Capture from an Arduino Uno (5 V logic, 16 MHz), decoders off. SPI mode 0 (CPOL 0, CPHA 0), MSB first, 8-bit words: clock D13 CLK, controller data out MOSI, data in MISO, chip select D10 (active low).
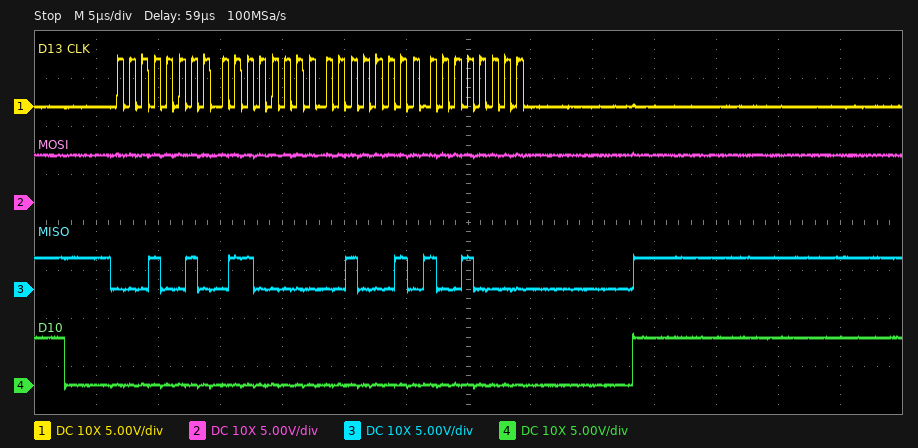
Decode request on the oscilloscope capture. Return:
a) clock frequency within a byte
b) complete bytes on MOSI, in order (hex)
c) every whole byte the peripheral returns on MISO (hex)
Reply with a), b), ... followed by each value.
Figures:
a) 1 MHz
b) 0xFF 0xFF 0xFF 0xFF
c) 0x12 0x60 0x22 0x90
